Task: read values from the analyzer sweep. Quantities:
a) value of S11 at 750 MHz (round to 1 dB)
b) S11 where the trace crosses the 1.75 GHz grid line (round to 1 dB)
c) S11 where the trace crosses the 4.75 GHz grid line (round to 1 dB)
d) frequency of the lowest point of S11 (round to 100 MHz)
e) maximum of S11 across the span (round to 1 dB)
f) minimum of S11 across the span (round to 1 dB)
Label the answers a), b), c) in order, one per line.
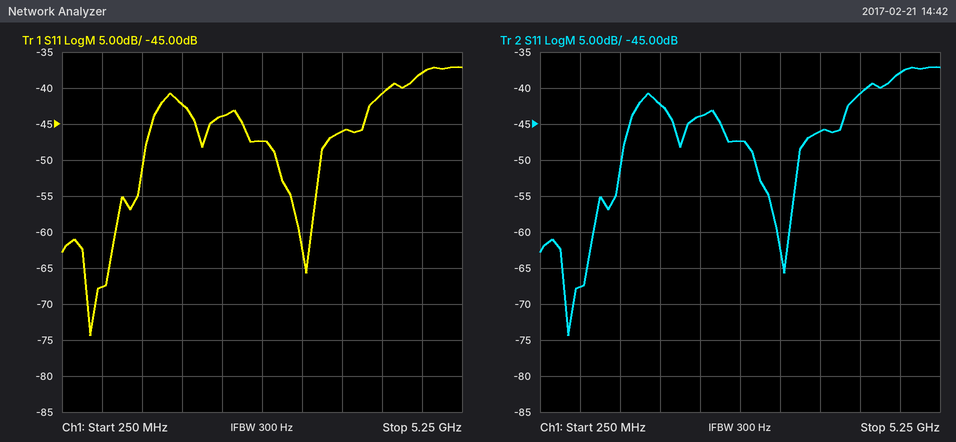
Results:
a) -68 dB
b) -42 dB
c) -38 dB
d) 600 MHz
e) -37 dB
f) -74 dB
